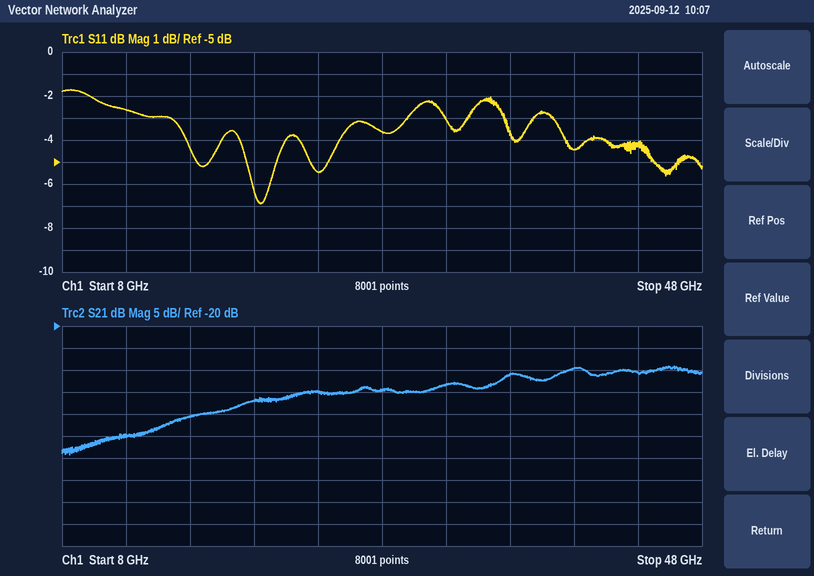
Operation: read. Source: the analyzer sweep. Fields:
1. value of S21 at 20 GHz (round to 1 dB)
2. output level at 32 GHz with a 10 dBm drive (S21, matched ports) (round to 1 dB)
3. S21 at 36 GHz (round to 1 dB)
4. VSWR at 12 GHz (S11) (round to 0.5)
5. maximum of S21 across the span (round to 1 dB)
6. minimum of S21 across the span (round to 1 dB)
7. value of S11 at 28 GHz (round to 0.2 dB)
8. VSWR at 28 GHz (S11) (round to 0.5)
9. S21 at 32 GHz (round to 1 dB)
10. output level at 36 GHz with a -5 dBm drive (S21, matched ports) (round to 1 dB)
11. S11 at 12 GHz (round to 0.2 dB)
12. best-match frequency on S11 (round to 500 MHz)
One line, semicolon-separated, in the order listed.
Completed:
-37 dB; -23 dBm; -31 dB; 6.5; -29 dB; -49 dB; -3.6 dB; 5.0; -33 dB; -36 dBm; -2.6 dB; 20.5 GHz
